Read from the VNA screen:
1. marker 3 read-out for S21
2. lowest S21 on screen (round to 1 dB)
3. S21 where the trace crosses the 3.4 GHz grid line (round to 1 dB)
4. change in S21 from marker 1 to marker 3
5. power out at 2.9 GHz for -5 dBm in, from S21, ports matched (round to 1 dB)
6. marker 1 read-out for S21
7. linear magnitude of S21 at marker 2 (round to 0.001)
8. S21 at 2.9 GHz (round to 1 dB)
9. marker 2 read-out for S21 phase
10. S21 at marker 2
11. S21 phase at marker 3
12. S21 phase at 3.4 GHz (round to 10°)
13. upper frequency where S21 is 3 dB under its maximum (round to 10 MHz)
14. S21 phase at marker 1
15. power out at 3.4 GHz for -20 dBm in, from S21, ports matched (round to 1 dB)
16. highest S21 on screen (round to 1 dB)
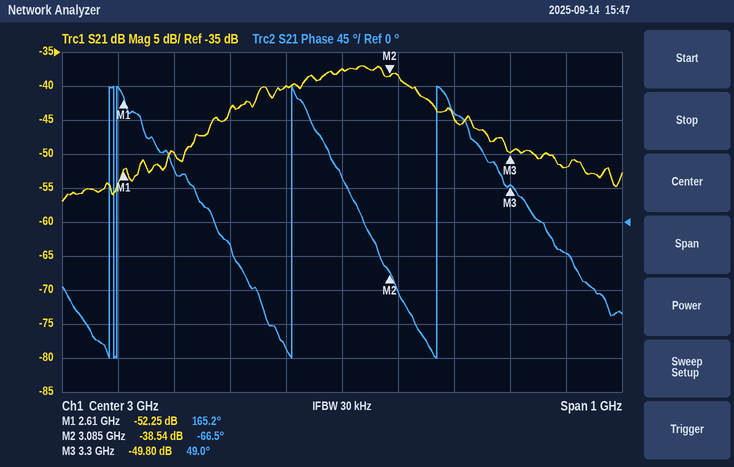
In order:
-49.80 dB
-57 dB
-52 dB
2.45 dB
-45 dBm
-52.25 dB
0.012
-40 dB
-66.5°
-38.54 dB
49.0°
-40°
3.12 GHz
165.2°
-72 dBm
-37 dB
